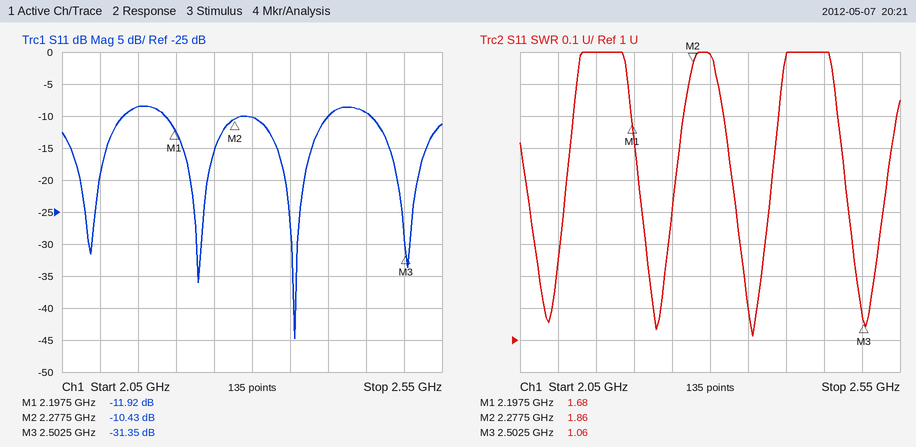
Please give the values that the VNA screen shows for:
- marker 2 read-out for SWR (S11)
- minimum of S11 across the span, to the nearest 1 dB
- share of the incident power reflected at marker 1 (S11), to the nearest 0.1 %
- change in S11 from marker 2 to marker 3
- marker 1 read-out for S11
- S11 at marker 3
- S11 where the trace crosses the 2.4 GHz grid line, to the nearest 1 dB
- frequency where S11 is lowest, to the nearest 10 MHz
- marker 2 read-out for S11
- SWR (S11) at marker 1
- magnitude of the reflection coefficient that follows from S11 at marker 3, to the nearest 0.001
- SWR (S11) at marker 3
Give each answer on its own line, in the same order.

1.86
-45 dB
6.4 %
-20.92 dB
-11.92 dB
-31.35 dB
-10 dB
2.36 GHz
-10.43 dB
1.68
0.027
1.06
